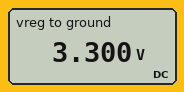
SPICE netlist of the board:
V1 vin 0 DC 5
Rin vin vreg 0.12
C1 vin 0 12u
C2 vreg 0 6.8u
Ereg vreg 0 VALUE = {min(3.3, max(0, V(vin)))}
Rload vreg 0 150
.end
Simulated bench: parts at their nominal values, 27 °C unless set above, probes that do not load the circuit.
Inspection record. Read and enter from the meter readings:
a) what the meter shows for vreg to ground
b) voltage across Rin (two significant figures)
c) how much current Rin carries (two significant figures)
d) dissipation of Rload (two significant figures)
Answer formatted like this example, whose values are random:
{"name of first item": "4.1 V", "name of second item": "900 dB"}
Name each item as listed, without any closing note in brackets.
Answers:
{"what the meter shows for vreg to ground": "3.300 V", "voltage across Rin": "1.7 V", "how much current Rin carries": "14 A", "dissipation of Rload": "73 mW"}
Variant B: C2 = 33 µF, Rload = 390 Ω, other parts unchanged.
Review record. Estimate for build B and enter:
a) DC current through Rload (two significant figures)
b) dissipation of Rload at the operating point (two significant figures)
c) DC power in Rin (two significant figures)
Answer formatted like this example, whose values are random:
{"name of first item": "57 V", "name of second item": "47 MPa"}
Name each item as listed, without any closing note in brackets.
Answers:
{"DC current through Rload": "8.5 mA", "dissipation of Rload at the operating point": "28 mW", "DC power in Rin": "24 W"}
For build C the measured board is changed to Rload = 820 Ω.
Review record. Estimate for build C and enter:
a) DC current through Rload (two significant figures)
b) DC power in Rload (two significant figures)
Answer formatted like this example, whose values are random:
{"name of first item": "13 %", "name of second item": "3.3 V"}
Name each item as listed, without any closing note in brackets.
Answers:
{"DC current through Rload": "4.0 mA", "DC power in Rload": "13 mW"}
